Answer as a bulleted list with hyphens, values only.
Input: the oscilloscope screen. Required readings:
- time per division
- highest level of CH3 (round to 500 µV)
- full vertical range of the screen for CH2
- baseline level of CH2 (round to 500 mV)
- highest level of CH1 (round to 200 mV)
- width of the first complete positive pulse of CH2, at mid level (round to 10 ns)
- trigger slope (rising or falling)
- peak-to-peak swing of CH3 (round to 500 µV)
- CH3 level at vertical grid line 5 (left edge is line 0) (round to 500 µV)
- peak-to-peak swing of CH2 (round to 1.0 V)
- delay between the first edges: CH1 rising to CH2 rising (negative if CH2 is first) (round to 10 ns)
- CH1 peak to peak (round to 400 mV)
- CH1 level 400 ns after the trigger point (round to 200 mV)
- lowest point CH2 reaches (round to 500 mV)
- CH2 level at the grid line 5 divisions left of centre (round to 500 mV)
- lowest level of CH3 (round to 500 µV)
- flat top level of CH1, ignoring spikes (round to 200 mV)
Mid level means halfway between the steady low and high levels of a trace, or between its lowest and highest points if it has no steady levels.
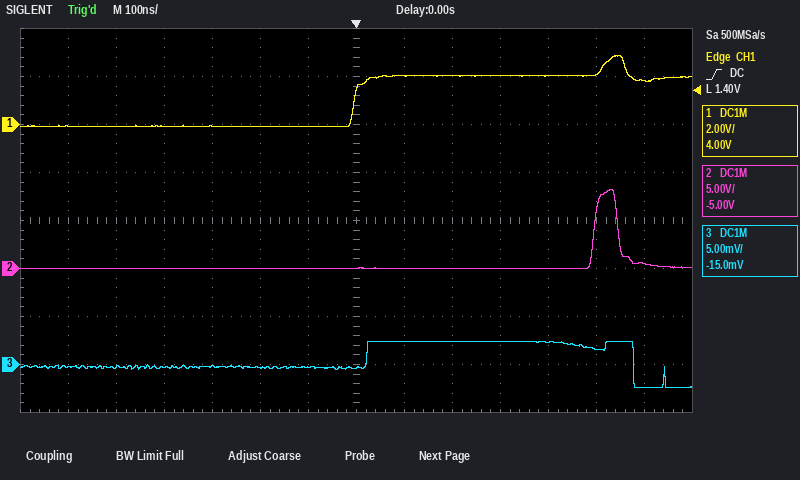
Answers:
- 100 ns
- 2.5 mV
- 40 V
- 0.0 V
- 2.8 V
- 50 ns
- rising
- 5.0 mV
- -500 µV
- 8.0 V
- +500 ns
- 2.8 V
- 2.0 V
- 0.0 V
- 0.0 V
- -2.5 mV
- 2.0 V
